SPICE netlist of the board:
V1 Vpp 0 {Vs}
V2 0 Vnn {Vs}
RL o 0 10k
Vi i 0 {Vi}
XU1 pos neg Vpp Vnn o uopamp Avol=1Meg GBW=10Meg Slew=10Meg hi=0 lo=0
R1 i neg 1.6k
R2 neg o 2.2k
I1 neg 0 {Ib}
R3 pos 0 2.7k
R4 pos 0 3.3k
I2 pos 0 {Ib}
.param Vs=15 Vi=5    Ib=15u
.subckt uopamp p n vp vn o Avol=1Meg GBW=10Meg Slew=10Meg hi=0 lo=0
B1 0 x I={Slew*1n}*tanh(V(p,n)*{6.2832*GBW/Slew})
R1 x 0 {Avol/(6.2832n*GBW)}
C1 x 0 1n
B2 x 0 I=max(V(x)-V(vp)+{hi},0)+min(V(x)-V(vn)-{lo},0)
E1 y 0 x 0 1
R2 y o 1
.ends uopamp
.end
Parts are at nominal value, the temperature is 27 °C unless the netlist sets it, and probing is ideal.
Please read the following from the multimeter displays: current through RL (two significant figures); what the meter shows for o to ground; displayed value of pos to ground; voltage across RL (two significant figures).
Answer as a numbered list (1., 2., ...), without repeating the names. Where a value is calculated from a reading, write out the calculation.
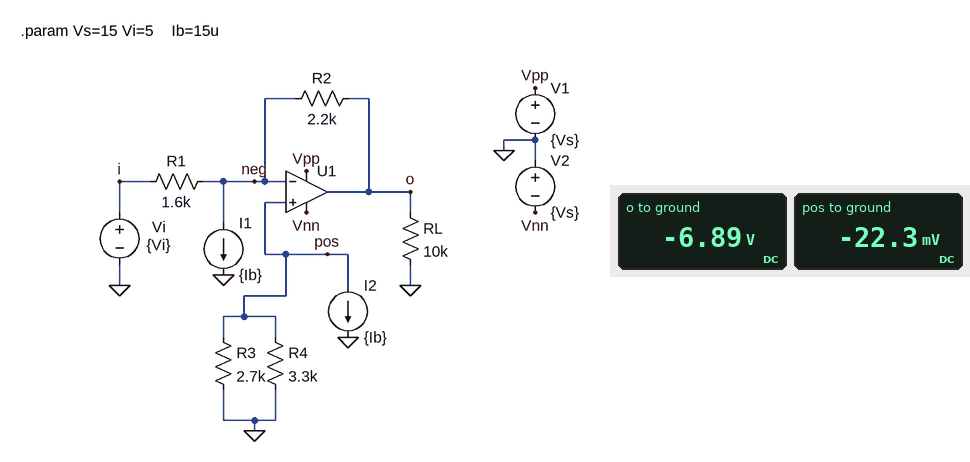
1. (0 V - (-6.89 V)) / 10 kΩ = 690 µA
2. -6.89 V
3. -22.3 mV
4. 0 V - (-6.89 V) = 6.9 V
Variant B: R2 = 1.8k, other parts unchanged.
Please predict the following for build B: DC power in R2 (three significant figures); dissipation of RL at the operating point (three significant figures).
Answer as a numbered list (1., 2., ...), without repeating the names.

1. 17.6 mW
2. 3.19 mW
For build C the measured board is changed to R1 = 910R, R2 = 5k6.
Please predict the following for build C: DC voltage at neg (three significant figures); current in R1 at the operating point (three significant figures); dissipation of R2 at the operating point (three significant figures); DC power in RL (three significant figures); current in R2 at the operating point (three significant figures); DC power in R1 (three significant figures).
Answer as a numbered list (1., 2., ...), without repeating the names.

1. 2.19 V
2. 3.09 mA
3. 52.8 mW
4. 22.5 mW
5. 3.07 mA
6. 8.67 mW
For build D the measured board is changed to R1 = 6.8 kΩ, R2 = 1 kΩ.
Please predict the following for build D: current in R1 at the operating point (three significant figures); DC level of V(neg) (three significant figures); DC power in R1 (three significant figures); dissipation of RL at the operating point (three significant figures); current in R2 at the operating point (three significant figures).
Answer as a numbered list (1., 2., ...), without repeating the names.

1. 739 µA
2. -22.3 mV
3. 3.71 mW
4. 55.6 µW
5. 724 µA
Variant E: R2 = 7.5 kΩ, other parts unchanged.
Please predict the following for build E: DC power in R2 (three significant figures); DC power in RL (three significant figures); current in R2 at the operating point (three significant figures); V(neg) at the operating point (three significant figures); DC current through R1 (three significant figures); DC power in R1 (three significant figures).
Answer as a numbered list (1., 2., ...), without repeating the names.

1. 36.2 mW
2. 22.5 mW
3. 2.20 mA
4. 1.46 V
5. 2.21 mA
6. 7.82 mW
